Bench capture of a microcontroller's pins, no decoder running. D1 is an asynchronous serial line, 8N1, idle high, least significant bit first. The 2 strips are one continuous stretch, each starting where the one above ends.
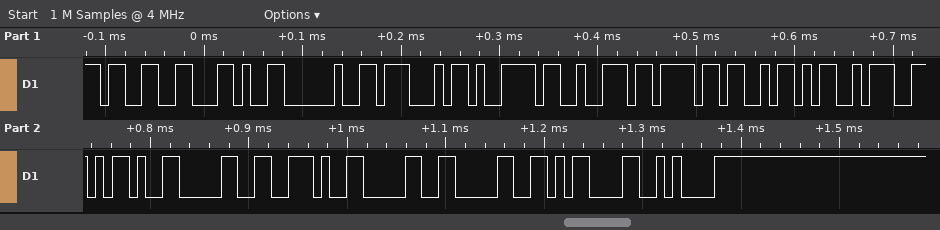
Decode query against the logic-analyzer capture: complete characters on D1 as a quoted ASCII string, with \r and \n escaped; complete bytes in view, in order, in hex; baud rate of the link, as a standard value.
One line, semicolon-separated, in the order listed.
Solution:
"3, GyroZ:-0.00\r\n"; 33 2C 20 47 79 72 6F 5A 3A 2D 30 2E 30 30 0D 0A; 115200 baud
